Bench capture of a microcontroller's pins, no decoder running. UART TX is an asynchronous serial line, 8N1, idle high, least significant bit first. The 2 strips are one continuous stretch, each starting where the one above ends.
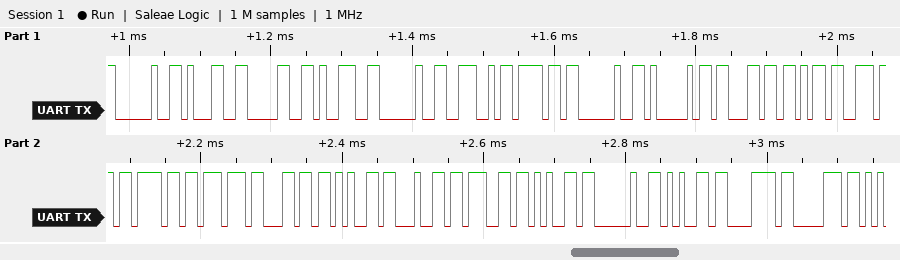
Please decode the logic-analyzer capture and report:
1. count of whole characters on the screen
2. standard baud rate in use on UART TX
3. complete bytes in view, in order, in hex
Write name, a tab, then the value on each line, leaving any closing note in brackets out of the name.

count of whole characters on the screen	23
standard baud rate in use on UART TX	115200 baud
complete bytes in view, in order, in hex	20 31 30 39 20 4E 6F 20 41 63 6B 6E 6F 77 6C 65 64 67 65 20 65 78 70
